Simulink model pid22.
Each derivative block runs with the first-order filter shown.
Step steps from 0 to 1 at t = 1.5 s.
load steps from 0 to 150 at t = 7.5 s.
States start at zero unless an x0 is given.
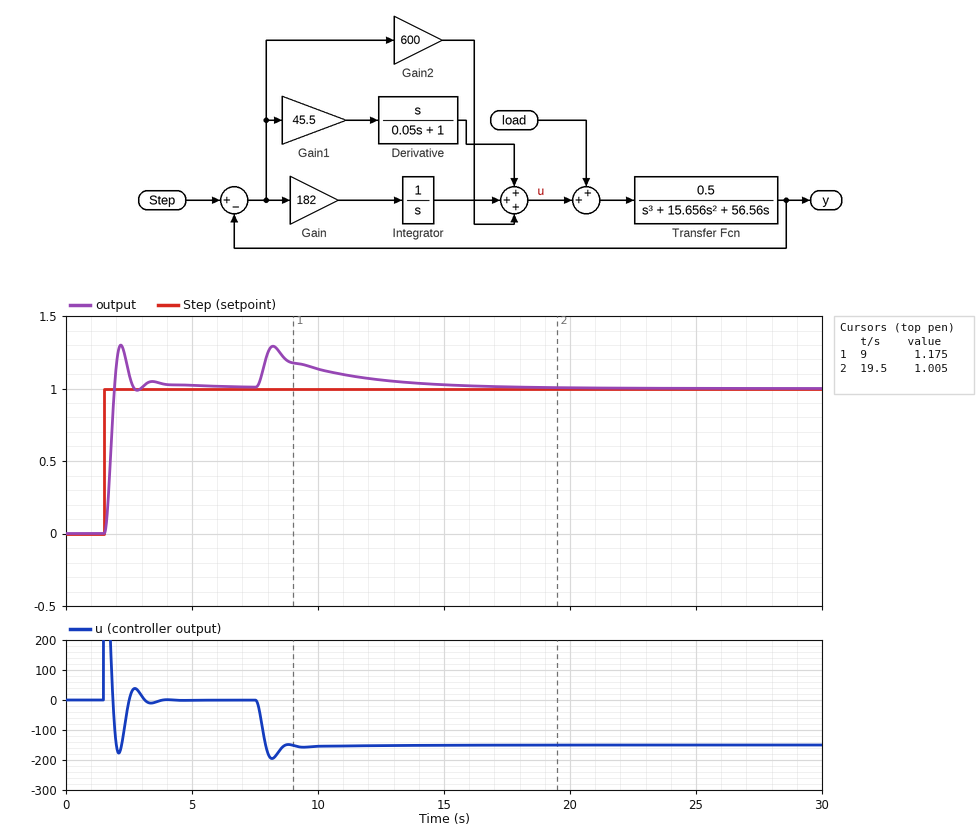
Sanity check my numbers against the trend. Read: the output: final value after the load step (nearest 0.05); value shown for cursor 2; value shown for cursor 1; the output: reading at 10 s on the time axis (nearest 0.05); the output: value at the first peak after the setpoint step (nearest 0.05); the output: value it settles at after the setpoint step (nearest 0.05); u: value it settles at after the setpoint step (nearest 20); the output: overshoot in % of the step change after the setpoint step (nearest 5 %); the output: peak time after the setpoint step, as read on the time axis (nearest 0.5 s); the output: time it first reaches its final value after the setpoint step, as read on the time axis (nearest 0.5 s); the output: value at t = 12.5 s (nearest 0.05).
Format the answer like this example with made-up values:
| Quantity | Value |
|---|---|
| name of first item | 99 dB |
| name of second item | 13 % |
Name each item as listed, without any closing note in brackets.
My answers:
| Quantity | Value |
|---|---|
| the output: final value after the load step | 1.00 |
| value shown for cursor 2 | 1.005 |
| value shown for cursor 1 | 1.175 |
| the output: reading at 10 s on the time axis | 1.15 |
| the output: value at the first peak after the setpoint step | 1.30 |
| the output: value it settles at after the setpoint step | 1.00 |
| u: value it settles at after the setpoint step | 0 |
| the output: overshoot in % of the step change after the setpoint step | 30 % |
| the output: peak time after the setpoint step, as read on the time axis | 2.0 s |
| the output: time it first reaches its final value after the setpoint step, as read on the time axis | 2.0 s |
| the output: value at t = 12.5 s | 1.05 |
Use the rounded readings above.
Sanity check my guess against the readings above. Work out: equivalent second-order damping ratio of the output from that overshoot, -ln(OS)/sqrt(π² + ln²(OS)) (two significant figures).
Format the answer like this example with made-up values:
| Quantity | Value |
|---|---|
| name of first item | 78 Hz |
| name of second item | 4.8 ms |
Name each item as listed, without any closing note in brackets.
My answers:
| Quantity | Value |
|---|---|
| equivalent second-order damping ratio of the output from that overshoot, -ln(OS)/sqrt(π² + ln²(OS)) | 0.36 |
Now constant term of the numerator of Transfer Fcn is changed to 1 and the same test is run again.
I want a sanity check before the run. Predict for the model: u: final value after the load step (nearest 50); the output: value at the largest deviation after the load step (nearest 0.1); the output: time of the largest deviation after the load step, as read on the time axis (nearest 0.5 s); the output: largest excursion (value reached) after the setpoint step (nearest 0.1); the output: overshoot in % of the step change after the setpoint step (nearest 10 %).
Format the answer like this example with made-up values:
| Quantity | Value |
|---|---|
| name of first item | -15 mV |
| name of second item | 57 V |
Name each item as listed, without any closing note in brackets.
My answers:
| Quantity | Value |
|---|---|
| u: final value after the load step | -150 |
| the output: value at the largest deviation after the load step | 1.3 |
| the output: time of the largest deviation after the load step, as read on the time axis | 8.0 s |
| the output: largest excursion (value reached) after the setpoint step | 1.5 |
| the output: overshoot in % of the step change after the setpoint step | 50 % |
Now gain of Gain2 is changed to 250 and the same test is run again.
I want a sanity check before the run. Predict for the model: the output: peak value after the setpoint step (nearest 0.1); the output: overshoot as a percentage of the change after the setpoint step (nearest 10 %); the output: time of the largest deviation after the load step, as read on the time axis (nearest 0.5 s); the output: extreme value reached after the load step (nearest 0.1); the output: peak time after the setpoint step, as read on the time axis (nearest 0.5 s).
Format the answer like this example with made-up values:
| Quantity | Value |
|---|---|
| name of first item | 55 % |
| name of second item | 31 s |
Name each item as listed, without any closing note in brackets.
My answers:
| Quantity | Value |
|---|---|
| the output: peak value after the setpoint step | 1.2 |
| the output: overshoot as a percentage of the change after the setpoint step | 20 % |
| the output: time of the largest deviation after the load step, as read on the time axis | 8.5 s |
| the output: extreme value reached after the load step | 1.5 |
| the output: peak time after the setpoint step, as read on the time axis | 3.0 s |
